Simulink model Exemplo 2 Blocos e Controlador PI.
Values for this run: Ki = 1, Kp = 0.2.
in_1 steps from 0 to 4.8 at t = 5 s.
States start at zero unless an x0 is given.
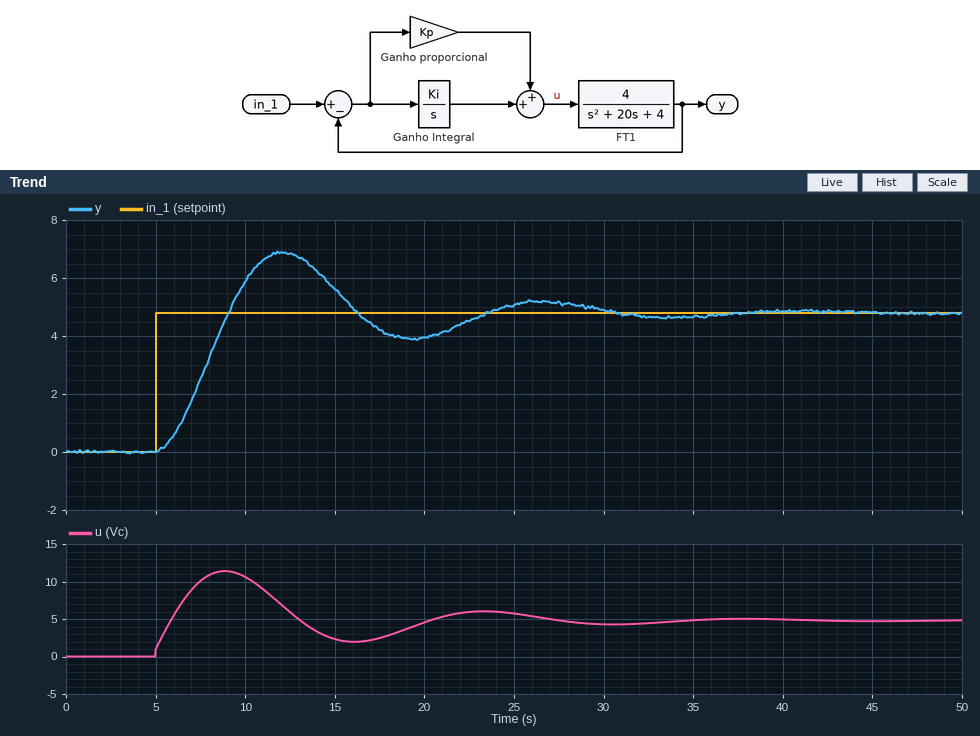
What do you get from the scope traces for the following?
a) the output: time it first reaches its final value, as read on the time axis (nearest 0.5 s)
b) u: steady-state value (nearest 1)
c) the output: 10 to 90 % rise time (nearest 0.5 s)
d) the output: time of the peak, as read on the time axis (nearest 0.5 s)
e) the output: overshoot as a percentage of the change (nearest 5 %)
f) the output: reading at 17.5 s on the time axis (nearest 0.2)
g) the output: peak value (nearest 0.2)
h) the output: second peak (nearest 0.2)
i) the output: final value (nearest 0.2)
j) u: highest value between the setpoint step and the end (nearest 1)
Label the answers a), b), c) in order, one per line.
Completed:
a) 9.0 s
b) 5
c) 3.0 s
d) 12.0 s
e) 45 %
f) 4.2
g) 6.8
h) 5.2
i) 4.8
j) 11
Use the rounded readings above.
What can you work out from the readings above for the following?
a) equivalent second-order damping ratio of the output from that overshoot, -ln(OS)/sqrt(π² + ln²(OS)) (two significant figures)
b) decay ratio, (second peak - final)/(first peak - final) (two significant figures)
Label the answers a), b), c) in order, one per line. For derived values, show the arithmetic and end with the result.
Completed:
a) ln(0.45) = -0.799; 0.799 / sqrt(9.870 + 0.638) = 0.25
b) (5.2 - 4.8) / (6.8 - 4.8) = 0.20
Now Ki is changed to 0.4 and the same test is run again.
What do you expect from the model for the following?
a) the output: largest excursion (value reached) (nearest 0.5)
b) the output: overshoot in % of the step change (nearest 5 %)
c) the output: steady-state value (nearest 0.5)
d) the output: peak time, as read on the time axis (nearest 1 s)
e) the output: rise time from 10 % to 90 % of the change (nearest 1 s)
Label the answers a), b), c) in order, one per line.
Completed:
a) 6.0
b) 25 %
c) 5.0
d) 17 s
e) 5 s
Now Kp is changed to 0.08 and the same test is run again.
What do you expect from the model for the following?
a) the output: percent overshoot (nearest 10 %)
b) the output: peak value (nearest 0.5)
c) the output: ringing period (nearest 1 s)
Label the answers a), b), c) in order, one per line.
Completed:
a) 50 %
b) 7.0
c) 14 s
